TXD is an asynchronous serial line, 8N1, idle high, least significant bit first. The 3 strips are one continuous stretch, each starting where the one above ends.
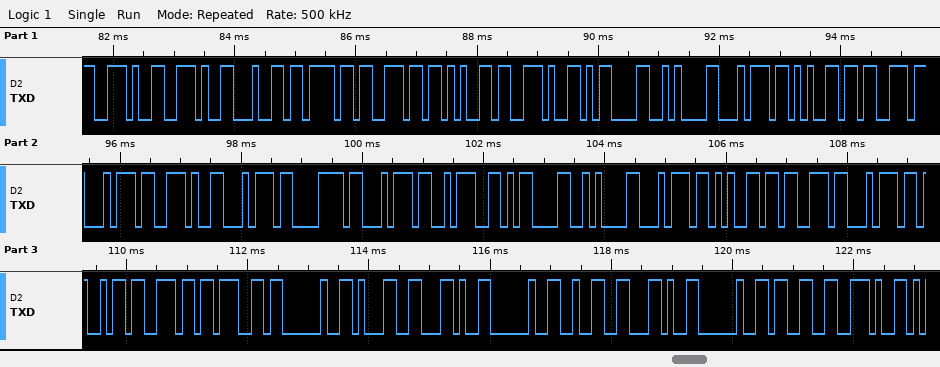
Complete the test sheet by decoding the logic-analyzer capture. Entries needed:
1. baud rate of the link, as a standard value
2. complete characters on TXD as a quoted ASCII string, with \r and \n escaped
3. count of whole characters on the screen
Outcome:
9600 baud
"..done.\r\ntest.txt:\r\ntesting 1, 2, 3."
36
